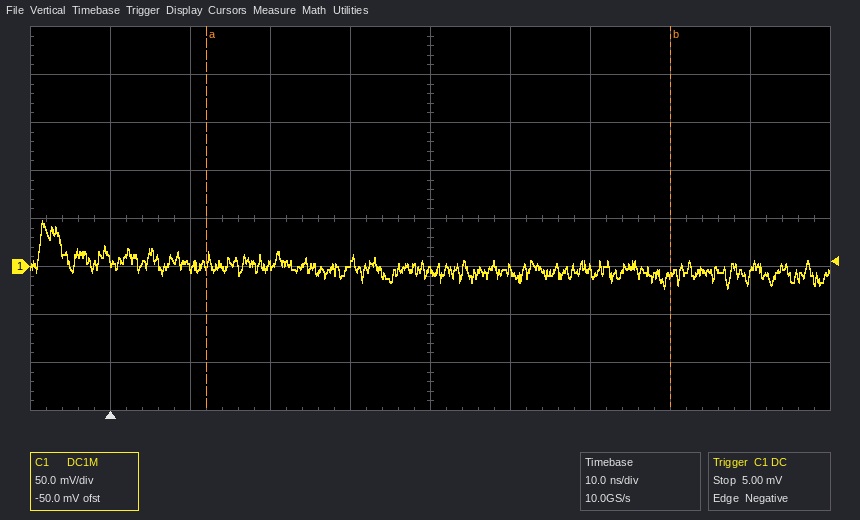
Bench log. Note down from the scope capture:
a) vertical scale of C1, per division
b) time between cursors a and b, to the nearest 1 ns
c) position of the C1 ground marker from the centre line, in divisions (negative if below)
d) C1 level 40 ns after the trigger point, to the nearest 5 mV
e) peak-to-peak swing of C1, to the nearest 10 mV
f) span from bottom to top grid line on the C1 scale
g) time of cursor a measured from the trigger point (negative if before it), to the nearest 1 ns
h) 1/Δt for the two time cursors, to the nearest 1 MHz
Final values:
50 mV
58 ns
-1.0 div
-5 mV
70 mV
400 mV
+12 ns
17 MHz
